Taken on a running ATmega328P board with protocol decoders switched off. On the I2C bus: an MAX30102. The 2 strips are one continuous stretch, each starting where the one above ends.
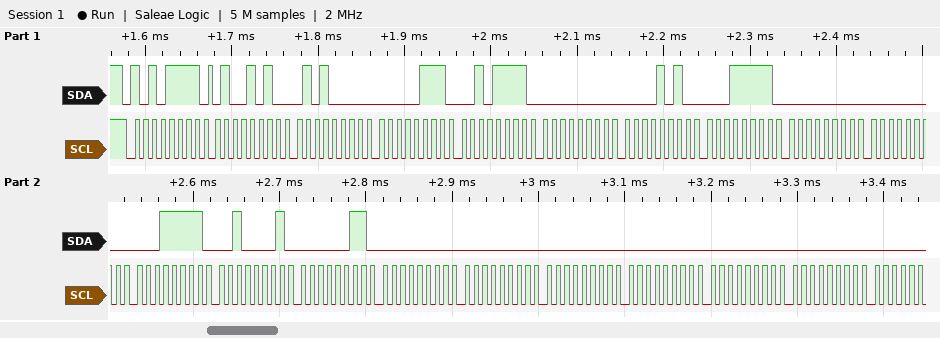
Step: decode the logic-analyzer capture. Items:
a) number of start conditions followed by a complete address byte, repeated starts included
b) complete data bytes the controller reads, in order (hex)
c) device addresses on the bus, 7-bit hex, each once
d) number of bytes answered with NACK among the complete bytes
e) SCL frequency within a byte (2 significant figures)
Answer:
1
4A 50 07 2F 00 0A 1F 00 00 1F 21 03 00 00 00 00 00 00
0x57
0
100 kHz
